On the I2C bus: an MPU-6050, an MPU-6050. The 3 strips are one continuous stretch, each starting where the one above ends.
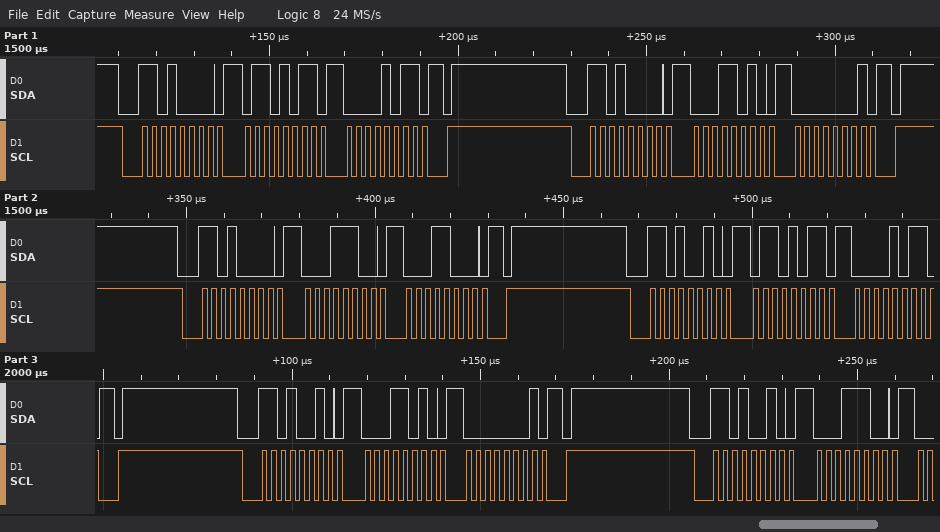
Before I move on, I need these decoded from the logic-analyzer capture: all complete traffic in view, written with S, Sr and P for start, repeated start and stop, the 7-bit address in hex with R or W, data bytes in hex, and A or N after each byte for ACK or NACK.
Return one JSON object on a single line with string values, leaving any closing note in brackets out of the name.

{"all complete traffic in view, written with S, Sr and P for start, repeated start and stop, the 7-bit address in hex with R or W, data bytes in hex, and A or N after each byte for ACK or NACK": "S 68W A 6B A 0B A P S 68W A 1A A 01 A P S 68W A 1C A 18 A P S 69W A 6B A 0B A P S 69W A 1A A 01 A P S 69W A 1C A"}
